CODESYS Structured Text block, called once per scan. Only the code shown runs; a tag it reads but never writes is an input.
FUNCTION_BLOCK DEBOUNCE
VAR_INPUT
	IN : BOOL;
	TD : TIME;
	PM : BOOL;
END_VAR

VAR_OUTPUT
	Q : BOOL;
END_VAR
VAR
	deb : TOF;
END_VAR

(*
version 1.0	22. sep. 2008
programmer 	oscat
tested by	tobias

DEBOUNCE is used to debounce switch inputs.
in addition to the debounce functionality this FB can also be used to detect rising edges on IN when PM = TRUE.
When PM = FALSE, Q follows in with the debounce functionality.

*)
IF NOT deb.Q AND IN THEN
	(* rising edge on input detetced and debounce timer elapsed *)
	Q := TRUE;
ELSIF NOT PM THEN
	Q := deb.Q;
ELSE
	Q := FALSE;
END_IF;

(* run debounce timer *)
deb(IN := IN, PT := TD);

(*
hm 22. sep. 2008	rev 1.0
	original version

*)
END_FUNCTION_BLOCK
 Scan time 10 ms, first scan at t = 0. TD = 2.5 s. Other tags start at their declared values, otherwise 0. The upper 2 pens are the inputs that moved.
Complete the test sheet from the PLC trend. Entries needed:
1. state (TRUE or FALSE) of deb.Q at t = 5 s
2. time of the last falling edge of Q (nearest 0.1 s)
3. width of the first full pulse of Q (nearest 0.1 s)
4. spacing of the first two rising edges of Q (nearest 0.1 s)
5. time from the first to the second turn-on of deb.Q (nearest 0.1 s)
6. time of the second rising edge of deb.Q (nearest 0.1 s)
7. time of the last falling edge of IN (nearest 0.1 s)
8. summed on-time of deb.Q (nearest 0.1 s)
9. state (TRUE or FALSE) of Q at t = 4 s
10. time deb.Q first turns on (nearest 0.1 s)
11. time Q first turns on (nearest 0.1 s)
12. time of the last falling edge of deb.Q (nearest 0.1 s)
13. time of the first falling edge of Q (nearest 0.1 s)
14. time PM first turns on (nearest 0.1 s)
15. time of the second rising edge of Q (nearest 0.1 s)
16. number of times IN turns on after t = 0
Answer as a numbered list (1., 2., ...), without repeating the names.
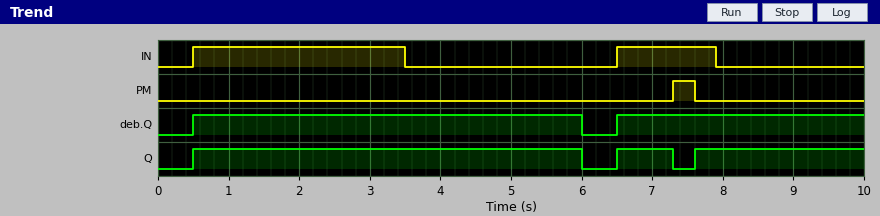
1. TRUE
2. 7.3 s
3. 5.5 s
4. 6.0 s
5. 6.0 s
6. 6.5 s
7. 7.9 s
8. 9.0 s
9. TRUE
10. 0.5 s
11. 0.5 s
12. 6.0 s
13. 6.0 s
14. 7.3 s
15. 6.5 s
16. 2
